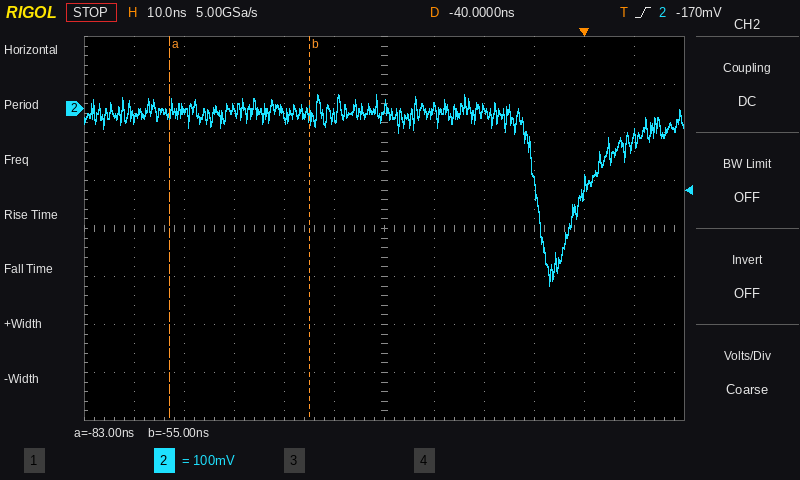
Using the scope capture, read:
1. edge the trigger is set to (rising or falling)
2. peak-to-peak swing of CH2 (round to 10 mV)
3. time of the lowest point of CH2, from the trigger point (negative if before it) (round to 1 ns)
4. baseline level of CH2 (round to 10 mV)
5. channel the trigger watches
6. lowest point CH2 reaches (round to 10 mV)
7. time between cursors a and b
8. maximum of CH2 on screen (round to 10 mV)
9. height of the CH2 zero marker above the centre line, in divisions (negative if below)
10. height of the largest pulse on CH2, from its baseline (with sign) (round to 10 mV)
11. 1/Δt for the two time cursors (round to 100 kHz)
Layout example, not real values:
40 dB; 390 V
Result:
rising; 400 mV; -7 ns; -10 mV; CH2; -370 mV; 28 ns; 30 mV; +2.5 div; -360 mV; 35.7 MHz
